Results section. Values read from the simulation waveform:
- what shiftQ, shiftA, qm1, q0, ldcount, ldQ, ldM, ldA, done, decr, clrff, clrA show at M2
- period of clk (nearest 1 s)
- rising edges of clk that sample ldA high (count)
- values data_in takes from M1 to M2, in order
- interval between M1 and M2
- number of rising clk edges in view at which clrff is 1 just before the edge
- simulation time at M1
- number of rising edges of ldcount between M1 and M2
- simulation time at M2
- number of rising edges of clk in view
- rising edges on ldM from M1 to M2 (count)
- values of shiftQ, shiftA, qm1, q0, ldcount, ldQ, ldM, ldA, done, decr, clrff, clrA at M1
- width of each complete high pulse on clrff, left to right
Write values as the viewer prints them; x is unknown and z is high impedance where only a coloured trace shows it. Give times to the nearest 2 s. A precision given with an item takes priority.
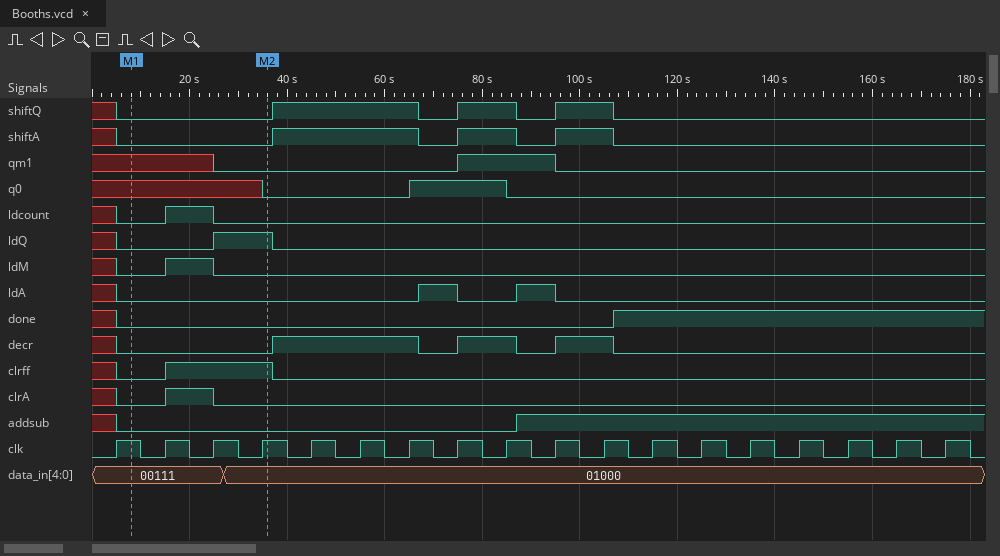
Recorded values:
shiftQ=0, shiftA=0, qm1=0, q0=0, ldcount=0, ldQ=1, ldM=0, ldA=0, done=0, decr=0, clrff=1, clrA=0
10 s
2
00111, 01000
28 s
2
8 s
1
36 s
18
1
shiftQ=0, shiftA=0, qm1=x, q0=x, ldcount=0, ldQ=0, ldM=0, ldA=0, done=0, decr=0, clrff=0, clrA=0
22 s
